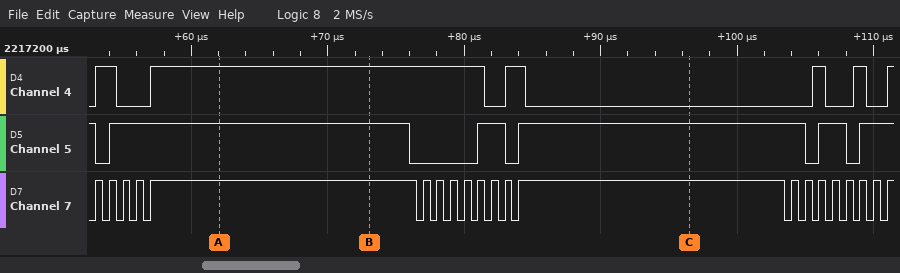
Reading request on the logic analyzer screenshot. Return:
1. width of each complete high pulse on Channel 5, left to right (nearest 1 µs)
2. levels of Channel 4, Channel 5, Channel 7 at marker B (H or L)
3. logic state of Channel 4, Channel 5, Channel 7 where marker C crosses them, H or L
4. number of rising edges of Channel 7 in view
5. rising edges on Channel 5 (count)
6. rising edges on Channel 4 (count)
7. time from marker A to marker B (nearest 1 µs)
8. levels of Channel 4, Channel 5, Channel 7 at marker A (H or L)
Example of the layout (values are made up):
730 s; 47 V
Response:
22 µs, 2 µs, 21 µs, 2 µs; Channel 4=H, Channel 5=H, Channel 7=H; Channel 4=L, Channel 5=H, Channel 7=H; 21; 5; 6; 11 µs; Channel 4=H, Channel 5=H, Channel 7=H
